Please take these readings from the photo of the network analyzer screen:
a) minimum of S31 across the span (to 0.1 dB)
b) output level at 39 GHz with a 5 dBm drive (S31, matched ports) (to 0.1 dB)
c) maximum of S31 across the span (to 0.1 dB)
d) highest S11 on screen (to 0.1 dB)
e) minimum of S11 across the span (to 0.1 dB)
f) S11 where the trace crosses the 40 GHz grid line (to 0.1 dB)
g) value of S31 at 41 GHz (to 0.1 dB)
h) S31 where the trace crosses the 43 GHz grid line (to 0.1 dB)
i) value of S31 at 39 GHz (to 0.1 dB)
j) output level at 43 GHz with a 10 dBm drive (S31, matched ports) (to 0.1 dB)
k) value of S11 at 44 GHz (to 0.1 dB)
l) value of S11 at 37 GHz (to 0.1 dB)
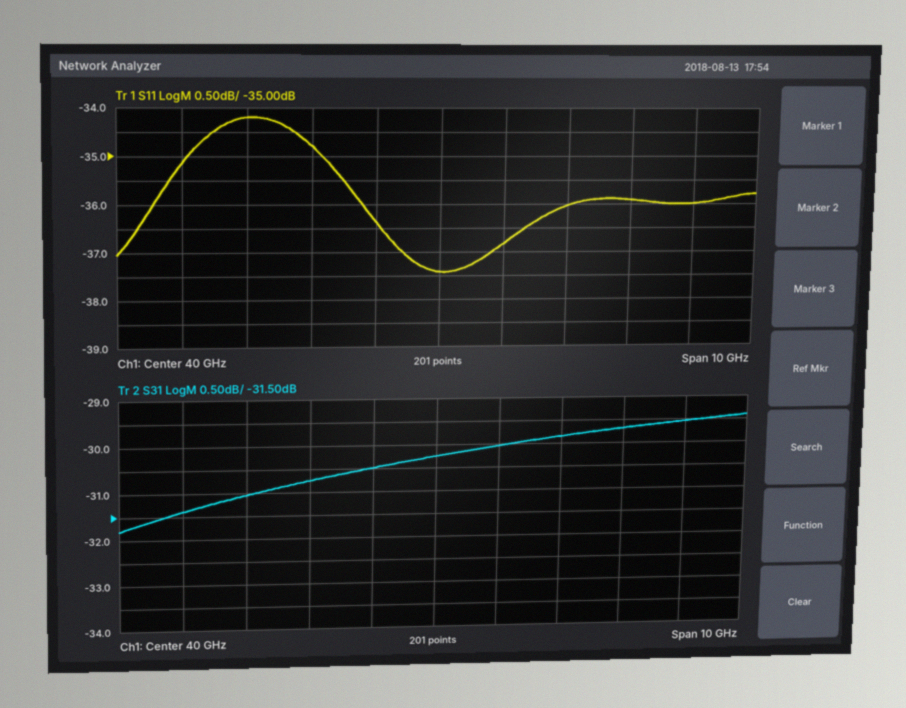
-31.8 dB
-25.5 dBm
-29.4 dB
-34.2 dB
-37.4 dB
-37.4 dB
-30.0 dB
-29.7 dB
-30.5 dB
-19.7 dBm
-36.0 dB
-34.2 dB
